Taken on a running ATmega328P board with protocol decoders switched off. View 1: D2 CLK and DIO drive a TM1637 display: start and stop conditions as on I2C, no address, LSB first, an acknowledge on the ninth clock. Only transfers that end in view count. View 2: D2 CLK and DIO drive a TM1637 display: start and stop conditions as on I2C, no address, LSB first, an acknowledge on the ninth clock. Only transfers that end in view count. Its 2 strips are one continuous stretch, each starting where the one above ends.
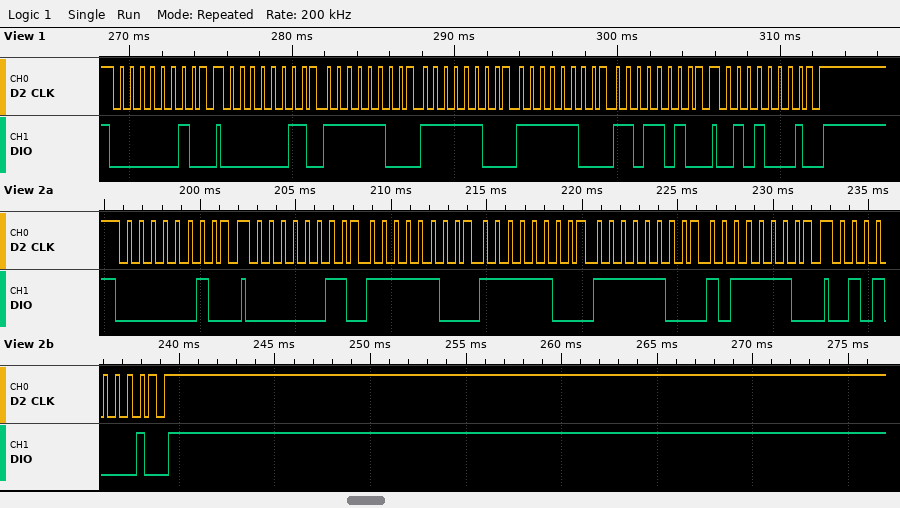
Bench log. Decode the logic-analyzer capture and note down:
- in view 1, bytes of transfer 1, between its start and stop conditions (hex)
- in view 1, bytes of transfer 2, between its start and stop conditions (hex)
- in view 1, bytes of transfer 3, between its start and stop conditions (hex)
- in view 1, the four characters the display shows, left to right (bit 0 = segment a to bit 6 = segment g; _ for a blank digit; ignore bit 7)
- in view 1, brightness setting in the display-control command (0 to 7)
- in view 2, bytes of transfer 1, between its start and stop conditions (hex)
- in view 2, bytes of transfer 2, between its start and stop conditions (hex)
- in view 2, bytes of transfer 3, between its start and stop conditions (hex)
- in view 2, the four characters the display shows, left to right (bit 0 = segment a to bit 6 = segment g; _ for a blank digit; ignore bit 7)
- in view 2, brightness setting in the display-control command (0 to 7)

40
C0 3F 3F 3F 5B
8A
0002
2
40
C0 3F 3F 3F 7D
8A
0006
2
